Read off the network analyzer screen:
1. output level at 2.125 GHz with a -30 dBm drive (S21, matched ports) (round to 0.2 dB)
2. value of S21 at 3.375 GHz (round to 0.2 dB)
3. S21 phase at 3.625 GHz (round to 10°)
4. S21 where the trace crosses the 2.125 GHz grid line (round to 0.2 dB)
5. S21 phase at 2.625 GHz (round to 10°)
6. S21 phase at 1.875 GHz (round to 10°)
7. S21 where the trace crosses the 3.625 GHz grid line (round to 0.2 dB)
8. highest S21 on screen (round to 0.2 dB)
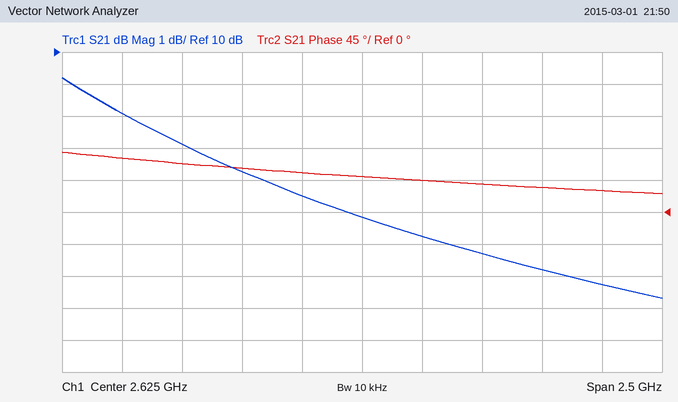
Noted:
-23.8 dBm
3.2 dB
30°
6.2 dB
50°
70°
2.8 dB
9.2 dB
